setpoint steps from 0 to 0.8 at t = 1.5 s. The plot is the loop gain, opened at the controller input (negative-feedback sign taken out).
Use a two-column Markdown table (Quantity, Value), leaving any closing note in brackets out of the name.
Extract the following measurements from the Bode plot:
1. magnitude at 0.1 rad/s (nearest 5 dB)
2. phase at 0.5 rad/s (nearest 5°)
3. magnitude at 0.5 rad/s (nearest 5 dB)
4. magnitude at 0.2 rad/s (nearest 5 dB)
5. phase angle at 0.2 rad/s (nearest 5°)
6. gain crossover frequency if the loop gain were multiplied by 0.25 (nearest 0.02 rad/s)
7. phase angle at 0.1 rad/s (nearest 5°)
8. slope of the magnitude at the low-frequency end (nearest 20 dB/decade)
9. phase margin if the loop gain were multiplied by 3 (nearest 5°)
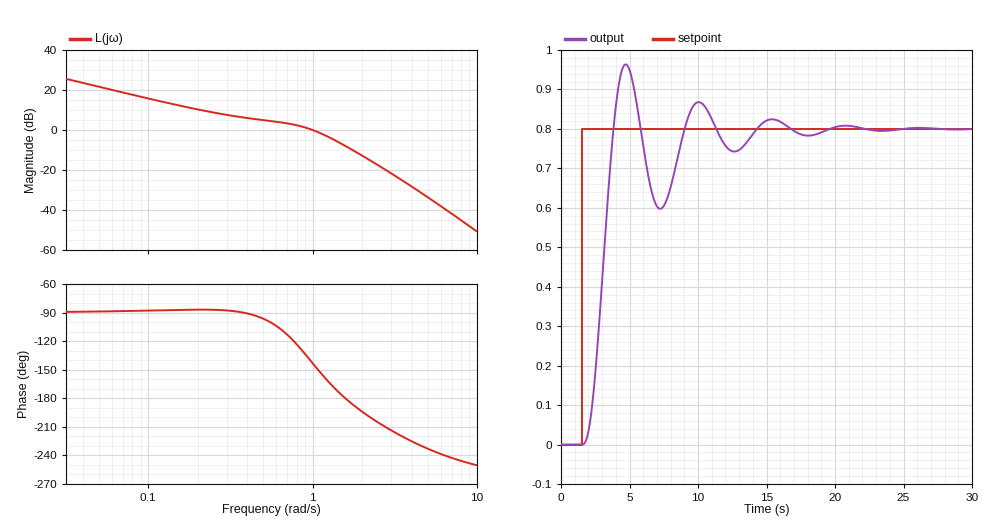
| Quantity | Value |
|---|---|
| magnitude at 0.1 rad/s | 15 dB |
| phase at 0.5 rad/s | -95° |
| magnitude at 0.5 rad/s | 5 dB |
| magnitude at 0.2 rad/s | 10 dB |
| phase angle at 0.2 rad/s | -85° |
| gain crossover frequency if the loop gain were multiplied by 0.25 | 0.16 rad/s |
| phase angle at 0.1 rad/s | -90° |
| slope of the magnitude at the low-frequency end | -20 dB/decade |
| phase margin if the loop gain were multiplied by 3 | -5° |
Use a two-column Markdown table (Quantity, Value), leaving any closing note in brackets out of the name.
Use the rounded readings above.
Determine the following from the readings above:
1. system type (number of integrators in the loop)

| Quantity | Value |
|---|---|
| system type | 1 |
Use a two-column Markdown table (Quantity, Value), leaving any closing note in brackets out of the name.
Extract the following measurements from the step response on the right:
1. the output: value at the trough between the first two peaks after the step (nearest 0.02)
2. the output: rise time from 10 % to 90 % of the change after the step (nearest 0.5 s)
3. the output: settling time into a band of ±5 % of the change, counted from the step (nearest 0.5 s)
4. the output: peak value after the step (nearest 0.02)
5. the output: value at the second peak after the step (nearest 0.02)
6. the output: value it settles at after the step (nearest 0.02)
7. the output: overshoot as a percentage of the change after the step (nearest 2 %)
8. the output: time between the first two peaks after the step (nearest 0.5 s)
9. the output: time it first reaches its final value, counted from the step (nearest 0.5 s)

| Quantity | Value |
|---|---|
| the output: value at the trough between the first two peaks after the step | 0.60 |
| the output: rise time from 10 % to 90 % of the change after the step | 1.5 s |
| the output: settling time into a band of ±5 % of the change, counted from the step | 12.0 s |
| the output: peak value after the step | 0.96 |
| the output: value at the second peak after the step | 0.86 |
| the output: value it settles at after the step | 0.80 |
| the output: overshoot as a percentage of the change after the step | 20 % |
| the output: time between the first two peaks after the step | 5.5 s |
| the output: time it first reaches its final value, counted from the step | 2.5 s |
